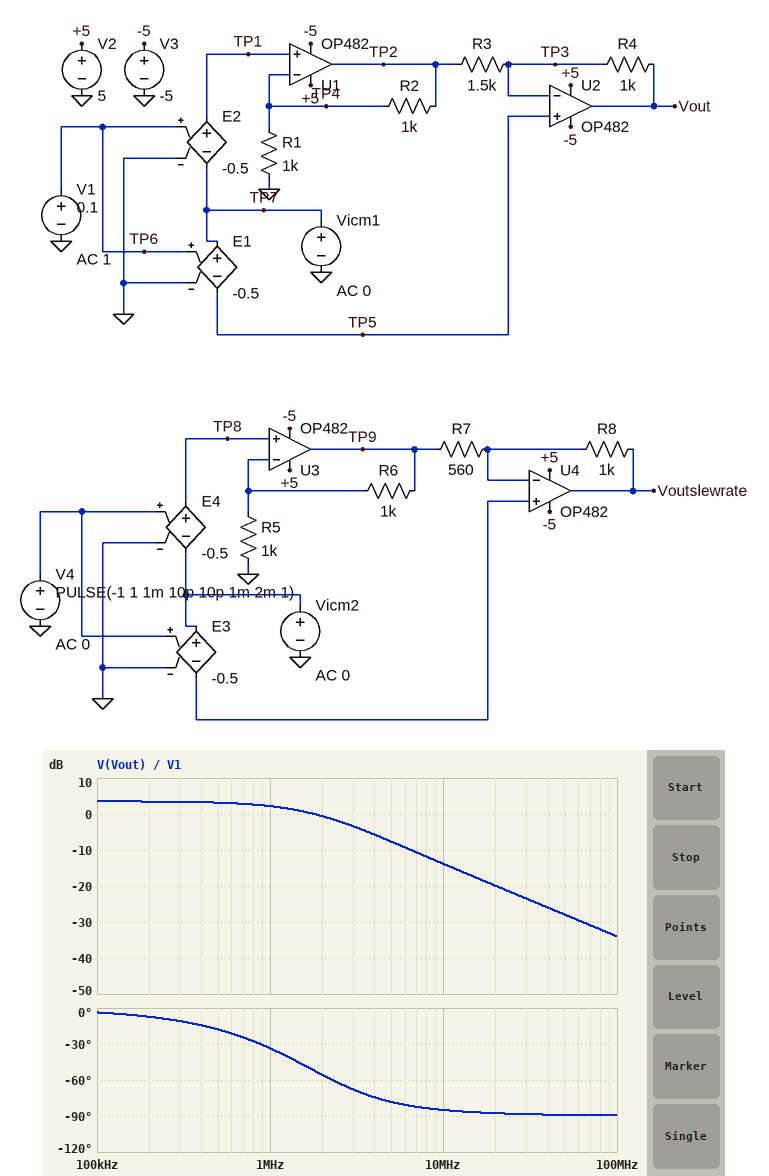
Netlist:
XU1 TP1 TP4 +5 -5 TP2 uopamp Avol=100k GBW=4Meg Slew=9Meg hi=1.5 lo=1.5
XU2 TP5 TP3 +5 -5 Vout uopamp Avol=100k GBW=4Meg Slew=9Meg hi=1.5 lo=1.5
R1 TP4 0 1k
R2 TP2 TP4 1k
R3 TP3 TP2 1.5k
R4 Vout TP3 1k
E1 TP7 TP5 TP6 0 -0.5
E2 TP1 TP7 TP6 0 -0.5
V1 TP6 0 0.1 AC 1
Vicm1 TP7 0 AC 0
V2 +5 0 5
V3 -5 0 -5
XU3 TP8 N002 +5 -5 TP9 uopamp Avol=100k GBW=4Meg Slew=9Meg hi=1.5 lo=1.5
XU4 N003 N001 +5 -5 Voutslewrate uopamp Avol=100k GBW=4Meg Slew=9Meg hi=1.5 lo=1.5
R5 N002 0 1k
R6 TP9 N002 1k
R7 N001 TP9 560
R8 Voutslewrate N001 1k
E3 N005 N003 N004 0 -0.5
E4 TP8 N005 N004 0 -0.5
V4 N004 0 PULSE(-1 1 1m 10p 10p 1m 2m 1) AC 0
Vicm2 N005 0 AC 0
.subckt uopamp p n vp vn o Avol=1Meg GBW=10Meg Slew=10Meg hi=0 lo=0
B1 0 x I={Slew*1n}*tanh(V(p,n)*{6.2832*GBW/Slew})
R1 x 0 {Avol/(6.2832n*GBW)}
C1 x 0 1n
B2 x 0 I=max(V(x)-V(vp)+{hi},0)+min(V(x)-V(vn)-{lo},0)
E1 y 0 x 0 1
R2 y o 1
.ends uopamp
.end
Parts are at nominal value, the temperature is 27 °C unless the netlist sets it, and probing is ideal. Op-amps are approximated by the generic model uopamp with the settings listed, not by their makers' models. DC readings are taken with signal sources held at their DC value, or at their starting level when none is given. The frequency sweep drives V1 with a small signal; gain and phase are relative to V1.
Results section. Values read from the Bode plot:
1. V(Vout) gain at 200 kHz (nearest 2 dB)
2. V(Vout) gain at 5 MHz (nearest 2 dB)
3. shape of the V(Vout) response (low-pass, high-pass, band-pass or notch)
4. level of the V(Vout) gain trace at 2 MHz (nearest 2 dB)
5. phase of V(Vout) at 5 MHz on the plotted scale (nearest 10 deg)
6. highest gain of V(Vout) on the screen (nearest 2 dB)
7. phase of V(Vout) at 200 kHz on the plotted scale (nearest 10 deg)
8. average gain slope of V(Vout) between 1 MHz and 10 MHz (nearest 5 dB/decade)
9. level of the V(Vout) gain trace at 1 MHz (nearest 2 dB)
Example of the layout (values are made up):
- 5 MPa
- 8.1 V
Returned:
- 4 dB
- -8 dB
- low-pass
- 0 dB
- -80 deg
- 4 dB
- -10 deg
- -15 dB/decade
- 2 dB
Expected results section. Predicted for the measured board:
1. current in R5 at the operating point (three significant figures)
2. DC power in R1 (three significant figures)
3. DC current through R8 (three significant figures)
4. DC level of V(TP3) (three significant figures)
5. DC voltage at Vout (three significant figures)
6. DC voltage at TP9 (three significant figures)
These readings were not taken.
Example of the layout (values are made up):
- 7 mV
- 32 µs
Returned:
- 500 µA
- 2.50 µW
- 2.68 mA
- 50.0 mV
- 150 mV
- 1.00 V
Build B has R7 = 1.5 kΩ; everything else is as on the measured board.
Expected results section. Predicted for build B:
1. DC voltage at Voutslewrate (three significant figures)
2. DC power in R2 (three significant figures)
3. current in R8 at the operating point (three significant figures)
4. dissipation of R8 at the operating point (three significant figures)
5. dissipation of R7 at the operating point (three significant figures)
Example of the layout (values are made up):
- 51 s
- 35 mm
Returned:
- -1.50 V
- 2.50 µW
- 1.00 mA
- 1.00 mW
- 1.50 mW
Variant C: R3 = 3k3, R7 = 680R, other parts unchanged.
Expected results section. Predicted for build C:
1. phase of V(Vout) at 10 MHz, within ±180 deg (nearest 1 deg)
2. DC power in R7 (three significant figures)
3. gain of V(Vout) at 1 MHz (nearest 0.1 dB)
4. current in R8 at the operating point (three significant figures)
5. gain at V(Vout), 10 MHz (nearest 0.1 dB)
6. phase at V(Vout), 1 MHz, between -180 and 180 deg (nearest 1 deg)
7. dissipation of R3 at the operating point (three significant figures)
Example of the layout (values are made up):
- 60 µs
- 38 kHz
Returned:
- -78 deg
- 3.31 mW
- -1.3 dB
- 2.21 mA
- -14.2 dB
- -26 deg
- 6.82 µW
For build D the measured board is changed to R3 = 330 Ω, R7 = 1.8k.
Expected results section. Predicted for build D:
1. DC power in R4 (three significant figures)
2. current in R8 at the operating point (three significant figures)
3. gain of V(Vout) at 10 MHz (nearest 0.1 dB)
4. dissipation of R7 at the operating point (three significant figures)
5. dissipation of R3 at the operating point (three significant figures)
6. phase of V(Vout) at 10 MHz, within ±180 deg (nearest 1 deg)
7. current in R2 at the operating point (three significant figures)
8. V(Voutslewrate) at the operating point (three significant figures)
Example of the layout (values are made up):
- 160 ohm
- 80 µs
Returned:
- 207 µW
- 833 µA
- -13.2 dB
- 1.25 mW
- 68.2 µW
- -100 deg
- 50.0 µA
- -1.33 V
